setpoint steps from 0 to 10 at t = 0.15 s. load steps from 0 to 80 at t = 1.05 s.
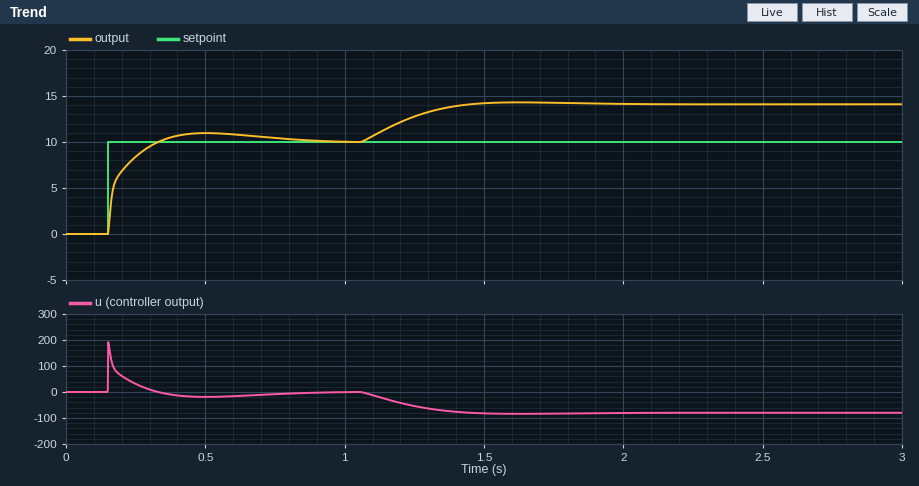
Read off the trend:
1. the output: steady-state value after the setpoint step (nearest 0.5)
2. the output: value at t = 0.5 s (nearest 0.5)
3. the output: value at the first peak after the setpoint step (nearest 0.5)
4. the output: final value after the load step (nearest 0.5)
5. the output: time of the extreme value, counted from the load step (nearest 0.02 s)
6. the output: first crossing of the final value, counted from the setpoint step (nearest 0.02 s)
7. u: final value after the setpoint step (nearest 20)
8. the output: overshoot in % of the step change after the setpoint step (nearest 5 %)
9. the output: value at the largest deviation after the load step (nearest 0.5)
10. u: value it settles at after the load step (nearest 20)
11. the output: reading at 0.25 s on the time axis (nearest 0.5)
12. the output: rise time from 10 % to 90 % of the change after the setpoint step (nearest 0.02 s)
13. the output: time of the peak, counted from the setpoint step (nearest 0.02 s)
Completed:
10.0
11.0
11.0
14.0
0.58 s
0.18 s
0
10 %
14.5
-80
8.5
0.12 s
0.36 s
